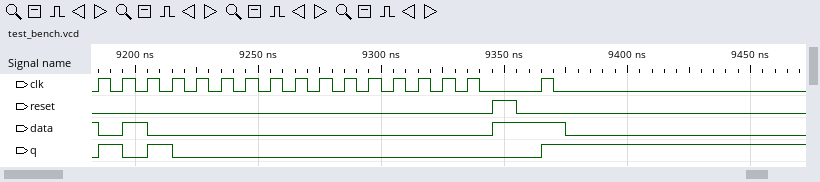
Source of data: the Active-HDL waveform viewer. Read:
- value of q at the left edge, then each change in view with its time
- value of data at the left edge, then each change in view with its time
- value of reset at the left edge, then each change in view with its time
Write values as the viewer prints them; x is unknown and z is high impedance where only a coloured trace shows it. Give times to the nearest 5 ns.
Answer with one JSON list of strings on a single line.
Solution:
["0, 1 at 9185 ns, 0 at 9195 ns, 1 at 9205 ns, 0 at 9215 ns, 1 at 9365 ns", "1, 0 at 9185 ns, 1 at 9195 ns, 0 at 9205 ns, 1 at 9345 ns, 0 at 9375 ns", "0, 1 at 9345 ns, 0 at 9355 ns"]
